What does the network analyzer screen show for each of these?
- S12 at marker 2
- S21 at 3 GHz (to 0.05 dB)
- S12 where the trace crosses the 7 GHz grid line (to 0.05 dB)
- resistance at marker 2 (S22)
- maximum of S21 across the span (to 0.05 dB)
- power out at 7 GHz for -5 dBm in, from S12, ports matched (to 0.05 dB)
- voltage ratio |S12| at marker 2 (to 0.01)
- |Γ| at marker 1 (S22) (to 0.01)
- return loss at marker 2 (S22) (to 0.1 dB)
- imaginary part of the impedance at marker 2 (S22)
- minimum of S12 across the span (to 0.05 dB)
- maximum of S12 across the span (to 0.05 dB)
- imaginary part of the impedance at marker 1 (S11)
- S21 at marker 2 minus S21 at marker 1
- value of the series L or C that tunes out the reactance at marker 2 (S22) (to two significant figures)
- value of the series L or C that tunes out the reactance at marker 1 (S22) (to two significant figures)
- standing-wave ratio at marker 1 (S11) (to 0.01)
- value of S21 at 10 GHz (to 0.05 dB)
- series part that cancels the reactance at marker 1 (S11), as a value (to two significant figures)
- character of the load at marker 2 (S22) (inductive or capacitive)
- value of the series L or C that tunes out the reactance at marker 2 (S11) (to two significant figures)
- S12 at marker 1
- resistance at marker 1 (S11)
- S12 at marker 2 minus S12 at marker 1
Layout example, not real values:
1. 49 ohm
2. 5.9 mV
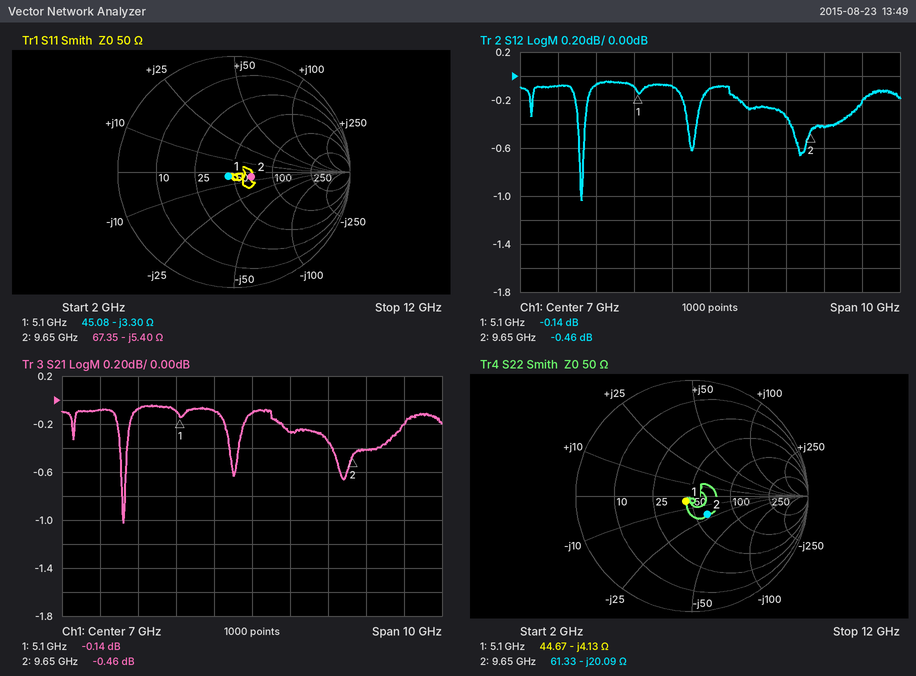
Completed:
1. -0.46 dB
2. -0.10 dB
3. -0.10 dB
4. 61.33 Ω
5. -0.05 dB
6. -5.10 dBm
7. 0.95
8. 0.07
9. 13.8 dB
10. -20.09 Ω
11. -1.05 dB
12. -0.05 dB
13. -3.30 Ω
14. -0.32 dB
15. 330 pH
16. 130 pH
17. 1.13
18. -0.40 dB
19. 100 pH
20. capacitive
21. 89 pH
22. -0.14 dB
23. 45.08 Ω
24. -0.32 dB
